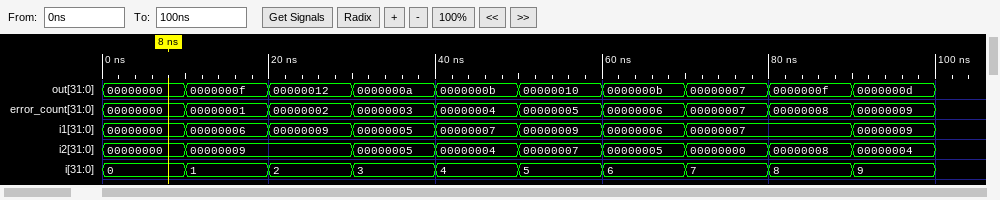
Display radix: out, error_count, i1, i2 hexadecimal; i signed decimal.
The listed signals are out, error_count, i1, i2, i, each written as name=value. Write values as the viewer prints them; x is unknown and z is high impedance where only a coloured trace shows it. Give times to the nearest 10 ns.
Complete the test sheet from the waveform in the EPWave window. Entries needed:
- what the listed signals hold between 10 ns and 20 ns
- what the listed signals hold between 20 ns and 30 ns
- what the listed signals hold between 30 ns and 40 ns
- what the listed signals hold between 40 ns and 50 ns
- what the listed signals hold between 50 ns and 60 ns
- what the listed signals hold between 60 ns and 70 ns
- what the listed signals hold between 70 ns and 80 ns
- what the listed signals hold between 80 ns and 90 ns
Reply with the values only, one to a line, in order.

out=0000000f, error_count=00000001, i1=00000006, i2=00000009, i=1
out=00000012, error_count=00000002, i1=00000009, i2=00000009, i=2
out=0000000a, error_count=00000003, i1=00000005, i2=00000005, i=3
out=0000000b, error_count=00000004, i1=00000007, i2=00000004, i=4
out=00000010, error_count=00000005, i1=00000009, i2=00000007, i=5
out=0000000b, error_count=00000006, i1=00000006, i2=00000005, i=6
out=00000007, error_count=00000007, i1=00000007, i2=00000000, i=7
out=0000000f, error_count=00000008, i1=00000007, i2=00000008, i=8
